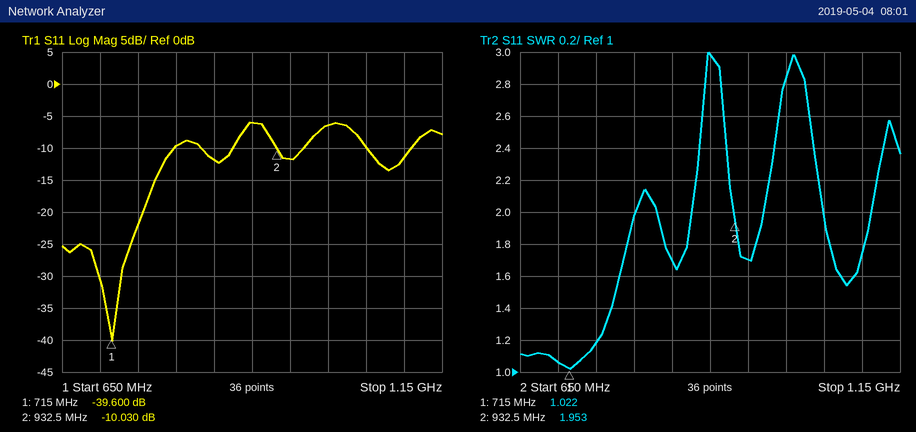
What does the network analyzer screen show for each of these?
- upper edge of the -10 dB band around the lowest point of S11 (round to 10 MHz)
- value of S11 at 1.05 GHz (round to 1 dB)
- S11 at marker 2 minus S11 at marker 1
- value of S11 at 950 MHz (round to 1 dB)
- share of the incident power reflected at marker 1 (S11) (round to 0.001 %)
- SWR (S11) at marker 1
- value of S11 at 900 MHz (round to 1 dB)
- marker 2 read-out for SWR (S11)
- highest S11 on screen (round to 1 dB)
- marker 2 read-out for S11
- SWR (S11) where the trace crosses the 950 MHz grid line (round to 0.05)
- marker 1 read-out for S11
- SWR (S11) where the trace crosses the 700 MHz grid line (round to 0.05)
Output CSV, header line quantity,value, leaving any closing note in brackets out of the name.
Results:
quantity,value
upper edge of the -10 dB band around the lowest point of S11,800 MHz
value of S11 at 1.05 GHz,-10 dB
S11 at marker 2 minus S11 at marker 1,29.570 dB
value of S11 at 950 MHz,-12 dB
share of the incident power reflected at marker 1 (S11),0.011 %
SWR (S11) at marker 1,1.022
value of S11 at 900 MHz,-6 dB
marker 2 read-out for SWR,1.953
highest S11 on screen,-6 dB
marker 2 read-out for S11,-10.030 dB
SWR (S11) where the trace crosses the 950 MHz grid line,1.70
marker 1 read-out for S11,-39.600 dB
SWR (S11) where the trace crosses the 700 MHz grid line,1.05
